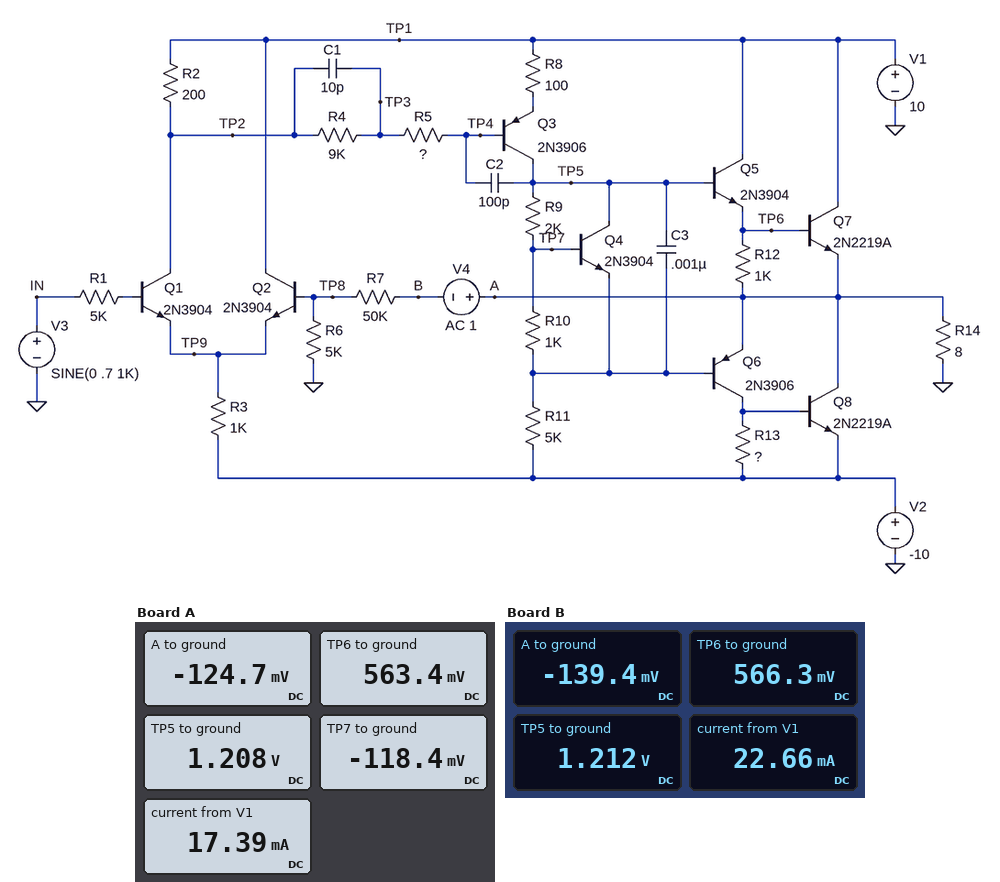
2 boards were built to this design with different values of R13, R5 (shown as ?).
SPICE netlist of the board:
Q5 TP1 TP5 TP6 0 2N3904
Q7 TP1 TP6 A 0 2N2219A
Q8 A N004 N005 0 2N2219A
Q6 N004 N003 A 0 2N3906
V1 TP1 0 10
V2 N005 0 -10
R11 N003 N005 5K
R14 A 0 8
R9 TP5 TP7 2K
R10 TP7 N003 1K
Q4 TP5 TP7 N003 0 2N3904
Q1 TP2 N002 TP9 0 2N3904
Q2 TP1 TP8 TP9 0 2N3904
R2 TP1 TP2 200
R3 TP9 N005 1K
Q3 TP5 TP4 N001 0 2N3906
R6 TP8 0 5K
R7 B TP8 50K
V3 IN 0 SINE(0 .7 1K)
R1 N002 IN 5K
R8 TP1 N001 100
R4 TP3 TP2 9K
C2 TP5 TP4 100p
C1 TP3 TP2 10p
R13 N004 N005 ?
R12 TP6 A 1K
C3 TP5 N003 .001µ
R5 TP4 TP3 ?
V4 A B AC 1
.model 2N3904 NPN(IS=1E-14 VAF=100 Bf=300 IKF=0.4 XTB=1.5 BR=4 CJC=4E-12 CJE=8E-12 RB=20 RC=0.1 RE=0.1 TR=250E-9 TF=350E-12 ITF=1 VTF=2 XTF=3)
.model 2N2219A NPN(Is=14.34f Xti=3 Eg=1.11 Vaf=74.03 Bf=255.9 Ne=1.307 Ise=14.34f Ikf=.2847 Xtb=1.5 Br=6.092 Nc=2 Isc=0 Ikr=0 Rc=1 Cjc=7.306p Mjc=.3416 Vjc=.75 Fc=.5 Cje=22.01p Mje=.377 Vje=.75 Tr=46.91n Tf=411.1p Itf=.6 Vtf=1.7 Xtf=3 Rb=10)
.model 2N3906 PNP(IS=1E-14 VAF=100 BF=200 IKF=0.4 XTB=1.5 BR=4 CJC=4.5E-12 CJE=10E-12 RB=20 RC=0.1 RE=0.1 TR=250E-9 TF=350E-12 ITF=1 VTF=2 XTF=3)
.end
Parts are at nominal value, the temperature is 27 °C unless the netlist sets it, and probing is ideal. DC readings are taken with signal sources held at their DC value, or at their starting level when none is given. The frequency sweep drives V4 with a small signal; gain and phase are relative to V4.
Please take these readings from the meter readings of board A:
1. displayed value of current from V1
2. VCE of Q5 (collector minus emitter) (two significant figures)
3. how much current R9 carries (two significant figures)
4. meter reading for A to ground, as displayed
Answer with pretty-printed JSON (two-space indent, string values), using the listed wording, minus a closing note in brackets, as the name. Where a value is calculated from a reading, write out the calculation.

{
  "displayed value of current from V1": "17.39 mA",
  "VCE of Q5 (collector minus emitter)": "10 V - 563.4 mV = 9.4 V",
  "how much current R9 carries": "(1.208 V - (-118.4 mV)) / 2 kΩ = 660 µA",
  "meter reading for A to ground, as displayed": "-124.7 mV"
}
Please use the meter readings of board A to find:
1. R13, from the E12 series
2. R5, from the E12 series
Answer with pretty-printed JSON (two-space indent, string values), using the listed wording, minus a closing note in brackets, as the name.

{
  "R13, from the E12 series": "820 Ω",
  "R5, from the E12 series": "820 Ω"
}
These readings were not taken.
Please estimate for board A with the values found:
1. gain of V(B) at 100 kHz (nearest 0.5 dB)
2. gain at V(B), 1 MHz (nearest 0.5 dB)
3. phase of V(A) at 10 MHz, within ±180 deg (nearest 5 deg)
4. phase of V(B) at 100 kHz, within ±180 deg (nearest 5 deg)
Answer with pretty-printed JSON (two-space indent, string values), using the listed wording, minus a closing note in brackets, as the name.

{
  "gain of V(B) at 100 kHz": "-1.5 dB",
  "gain at V(B), 1 MHz": "0 dB",
  "phase of V(A) at 10 MHz, within ±180 deg": "-170 deg",
  "phase of V(B) at 100 kHz, within ±180 deg": "-150 deg"
}
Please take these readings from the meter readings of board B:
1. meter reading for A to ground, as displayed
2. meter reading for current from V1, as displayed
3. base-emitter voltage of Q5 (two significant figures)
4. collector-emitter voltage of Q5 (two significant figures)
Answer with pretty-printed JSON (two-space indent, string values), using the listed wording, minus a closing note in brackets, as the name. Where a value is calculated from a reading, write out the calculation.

{
  "meter reading for A to ground, as displayed": "-139.4 mV",
  "meter reading for current from V1, as displayed": "22.66 mA",
  "base-emitter voltage of Q5": "1.212 V - 566.3 mV = 650 mV",
  "collector-emitter voltage of Q5": "10 V - 566.3 mV = 9.4 V"
}
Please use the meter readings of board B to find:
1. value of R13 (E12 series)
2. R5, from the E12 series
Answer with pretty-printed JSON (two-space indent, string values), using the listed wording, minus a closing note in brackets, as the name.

{
  "value of R13": "2.2 kΩ",
  "R5, from the E12 series": "1.5 kΩ"
}
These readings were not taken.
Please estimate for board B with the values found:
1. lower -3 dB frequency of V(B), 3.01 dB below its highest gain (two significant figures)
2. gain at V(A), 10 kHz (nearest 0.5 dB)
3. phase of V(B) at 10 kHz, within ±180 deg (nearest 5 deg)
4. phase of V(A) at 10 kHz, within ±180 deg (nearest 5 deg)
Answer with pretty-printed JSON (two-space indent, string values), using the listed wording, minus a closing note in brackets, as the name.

{
  "lower -3 dB frequency of V(B), 3.01 dB below its highest gain": "63 kHz",
  "gain at V(A), 10 kHz": "-1.0 dB",
  "phase of V(B) at 10 kHz, within ±180 deg": "-125 deg",
  "phase of V(A) at 10 kHz, within ±180 deg": "-10 deg"
}
